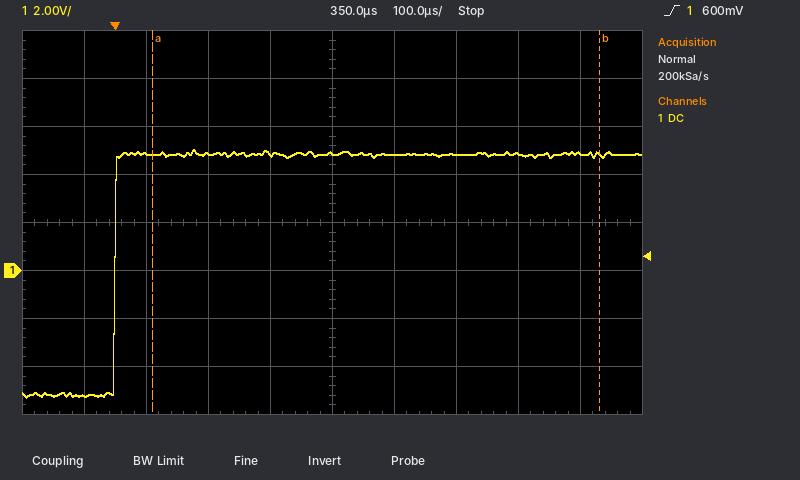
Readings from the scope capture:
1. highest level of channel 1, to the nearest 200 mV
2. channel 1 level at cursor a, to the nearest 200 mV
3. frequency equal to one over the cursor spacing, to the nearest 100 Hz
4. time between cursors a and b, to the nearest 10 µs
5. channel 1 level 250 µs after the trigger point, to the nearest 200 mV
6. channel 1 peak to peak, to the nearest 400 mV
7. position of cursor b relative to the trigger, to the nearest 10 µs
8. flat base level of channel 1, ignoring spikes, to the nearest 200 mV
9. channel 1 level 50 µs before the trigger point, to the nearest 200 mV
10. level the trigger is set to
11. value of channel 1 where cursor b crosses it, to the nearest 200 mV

5.0 V
4.8 V
1.4 kHz
720 µs
4.8 V
10.4 V
+780 µs
-5.2 V
-5.2 V
600 mV
4.8 V
